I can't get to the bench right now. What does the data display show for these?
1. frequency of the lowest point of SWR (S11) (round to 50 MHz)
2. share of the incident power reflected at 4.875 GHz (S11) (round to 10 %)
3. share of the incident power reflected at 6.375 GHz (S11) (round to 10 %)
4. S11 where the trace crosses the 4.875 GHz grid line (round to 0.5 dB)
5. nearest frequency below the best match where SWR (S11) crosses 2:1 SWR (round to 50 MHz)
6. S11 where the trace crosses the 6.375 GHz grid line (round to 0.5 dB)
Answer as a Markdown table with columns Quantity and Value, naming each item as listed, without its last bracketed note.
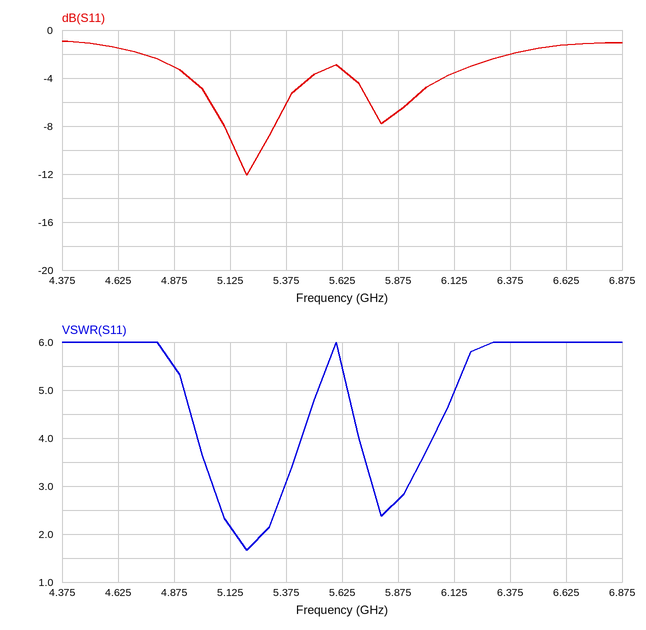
| Quantity | Value |
|---|---|
| frequency of the lowest point of SWR (S11) | 5.20 GHz |
| share of the incident power reflected at 4.875 GHz (S11) | 50 % |
| share of the incident power reflected at 6.375 GHz (S11) | 60 % |
| S11 where the trace crosses the 4.875 GHz grid line | -3.0 dB |
| nearest frequency below the best match where SWR (S11) crosses 2:1 SWR | 5.15 GHz |
| S11 where the trace crosses the 6.375 GHz grid line | -2.0 dB |
